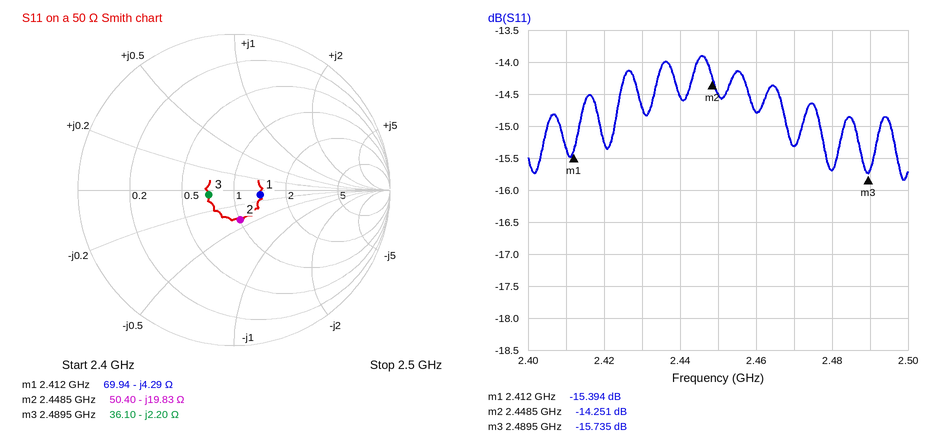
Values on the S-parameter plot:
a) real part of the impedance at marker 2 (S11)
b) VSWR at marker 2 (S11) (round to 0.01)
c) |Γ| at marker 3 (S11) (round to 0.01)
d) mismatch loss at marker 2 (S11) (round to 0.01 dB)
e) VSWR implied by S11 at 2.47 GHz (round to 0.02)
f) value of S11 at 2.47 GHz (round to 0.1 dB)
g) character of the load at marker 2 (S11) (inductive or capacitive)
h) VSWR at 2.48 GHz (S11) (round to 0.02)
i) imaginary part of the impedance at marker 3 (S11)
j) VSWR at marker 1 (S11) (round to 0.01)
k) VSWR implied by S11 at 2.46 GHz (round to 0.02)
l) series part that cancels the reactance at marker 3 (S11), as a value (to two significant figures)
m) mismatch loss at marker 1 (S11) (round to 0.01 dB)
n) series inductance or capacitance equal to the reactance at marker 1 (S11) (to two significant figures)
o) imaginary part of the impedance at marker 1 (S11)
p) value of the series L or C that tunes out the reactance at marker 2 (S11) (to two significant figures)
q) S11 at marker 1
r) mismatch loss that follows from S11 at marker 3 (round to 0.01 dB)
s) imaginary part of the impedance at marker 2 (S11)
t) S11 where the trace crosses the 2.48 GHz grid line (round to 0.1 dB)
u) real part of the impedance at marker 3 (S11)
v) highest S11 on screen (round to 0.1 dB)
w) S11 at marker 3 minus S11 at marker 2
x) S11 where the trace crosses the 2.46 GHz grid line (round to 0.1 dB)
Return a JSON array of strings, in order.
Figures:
["50.40 Ω", "1.48", "0.16", "0.17 dB", "1.42", "-15.3 dB", "capacitive", "1.40", "-2.20 Ω", "1.41", "1.44", "140 pH", "0.13 dB", "15 pF", "-4.29 Ω", "1.3 nH", "-15.394 dB", "0.12 dB", "-19.83 Ω", "-15.7 dB", "36.10 Ω", "-13.9 dB", "-1.484 dB", "-14.8 dB"]
